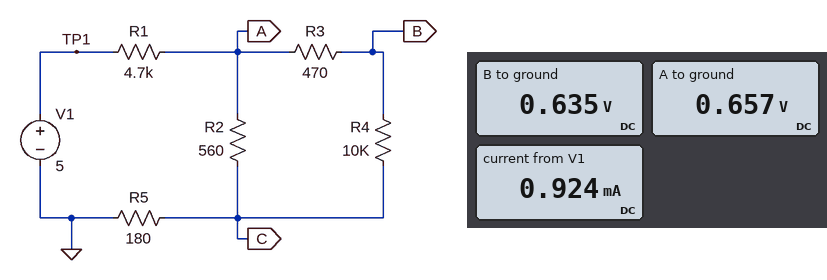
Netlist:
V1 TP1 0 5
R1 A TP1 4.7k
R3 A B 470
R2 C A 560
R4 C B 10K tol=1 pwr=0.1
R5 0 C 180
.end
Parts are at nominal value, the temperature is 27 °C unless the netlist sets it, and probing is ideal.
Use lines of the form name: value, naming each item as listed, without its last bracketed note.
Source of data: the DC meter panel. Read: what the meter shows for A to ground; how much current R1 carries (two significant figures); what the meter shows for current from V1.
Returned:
what the meter shows for A to ground: 0.657 V
how much current R1 carries: 920 µA
what the meter shows for current from V1: 0.924 mA
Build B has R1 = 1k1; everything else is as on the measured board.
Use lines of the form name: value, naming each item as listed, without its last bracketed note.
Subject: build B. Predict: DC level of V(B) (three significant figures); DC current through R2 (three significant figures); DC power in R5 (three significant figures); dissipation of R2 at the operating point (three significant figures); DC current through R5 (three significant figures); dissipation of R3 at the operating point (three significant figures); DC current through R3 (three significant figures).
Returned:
DC level of V(B): 1.90 V
DC current through R2: 2.62 mA
DC power in R5: 1.37 mW
dissipation of R2 at the operating point: 3.84 mW
DC current through R5: 2.76 mA
dissipation of R3 at the operating point: 9.23 µW
DC current through R3: 140 µA
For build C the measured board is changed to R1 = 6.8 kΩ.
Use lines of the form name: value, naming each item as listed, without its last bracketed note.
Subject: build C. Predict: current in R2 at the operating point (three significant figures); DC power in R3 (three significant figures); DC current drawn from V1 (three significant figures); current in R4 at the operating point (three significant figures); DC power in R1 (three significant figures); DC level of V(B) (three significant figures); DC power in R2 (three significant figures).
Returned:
current in R2 at the operating point: 632 µA
DC power in R3: 537 nW
DC current drawn from V1: 666 µA
current in R4 at the operating point: 33.8 µA
DC power in R1: 3.01 mW
DC level of V(B): 458 mV
DC power in R2: 224 µW
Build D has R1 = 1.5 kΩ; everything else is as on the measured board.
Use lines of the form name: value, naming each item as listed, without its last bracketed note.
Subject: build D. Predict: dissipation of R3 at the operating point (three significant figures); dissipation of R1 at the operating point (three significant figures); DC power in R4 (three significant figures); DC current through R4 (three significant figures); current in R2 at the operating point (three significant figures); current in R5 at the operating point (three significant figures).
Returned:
dissipation of R3 at the operating point: 6.19 µW
dissipation of R1 at the operating point: 7.67 mW
DC power in R4: 132 µW
DC current through R4: 115 µA
current in R2 at the operating point: 2.15 mA
current in R5 at the operating point: 2.26 mA
